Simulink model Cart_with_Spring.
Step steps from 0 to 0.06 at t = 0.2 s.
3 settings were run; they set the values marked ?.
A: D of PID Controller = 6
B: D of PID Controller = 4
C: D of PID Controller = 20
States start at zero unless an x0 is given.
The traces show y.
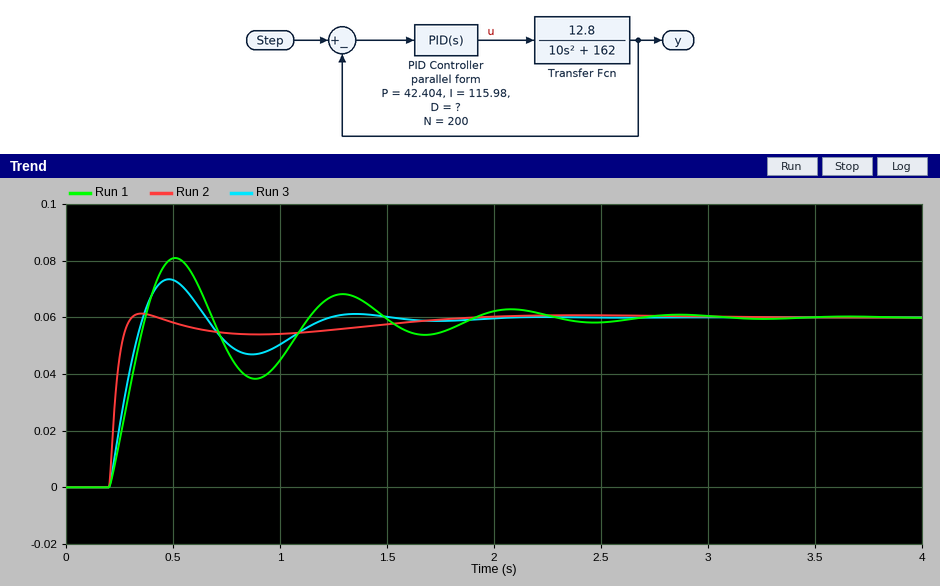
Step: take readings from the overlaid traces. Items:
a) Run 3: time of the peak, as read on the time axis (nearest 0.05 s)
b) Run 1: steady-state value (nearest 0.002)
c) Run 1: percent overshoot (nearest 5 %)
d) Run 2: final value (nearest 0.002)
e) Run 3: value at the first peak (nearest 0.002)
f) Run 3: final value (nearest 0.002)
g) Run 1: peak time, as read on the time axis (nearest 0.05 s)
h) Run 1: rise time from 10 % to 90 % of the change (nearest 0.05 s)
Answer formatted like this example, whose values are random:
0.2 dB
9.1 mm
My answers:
0.50 s
0.060
35 %
0.060
0.074
0.060
0.50 s
0.15 s
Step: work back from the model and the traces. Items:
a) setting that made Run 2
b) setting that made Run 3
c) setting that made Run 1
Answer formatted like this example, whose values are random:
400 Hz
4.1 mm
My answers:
C
A
B
